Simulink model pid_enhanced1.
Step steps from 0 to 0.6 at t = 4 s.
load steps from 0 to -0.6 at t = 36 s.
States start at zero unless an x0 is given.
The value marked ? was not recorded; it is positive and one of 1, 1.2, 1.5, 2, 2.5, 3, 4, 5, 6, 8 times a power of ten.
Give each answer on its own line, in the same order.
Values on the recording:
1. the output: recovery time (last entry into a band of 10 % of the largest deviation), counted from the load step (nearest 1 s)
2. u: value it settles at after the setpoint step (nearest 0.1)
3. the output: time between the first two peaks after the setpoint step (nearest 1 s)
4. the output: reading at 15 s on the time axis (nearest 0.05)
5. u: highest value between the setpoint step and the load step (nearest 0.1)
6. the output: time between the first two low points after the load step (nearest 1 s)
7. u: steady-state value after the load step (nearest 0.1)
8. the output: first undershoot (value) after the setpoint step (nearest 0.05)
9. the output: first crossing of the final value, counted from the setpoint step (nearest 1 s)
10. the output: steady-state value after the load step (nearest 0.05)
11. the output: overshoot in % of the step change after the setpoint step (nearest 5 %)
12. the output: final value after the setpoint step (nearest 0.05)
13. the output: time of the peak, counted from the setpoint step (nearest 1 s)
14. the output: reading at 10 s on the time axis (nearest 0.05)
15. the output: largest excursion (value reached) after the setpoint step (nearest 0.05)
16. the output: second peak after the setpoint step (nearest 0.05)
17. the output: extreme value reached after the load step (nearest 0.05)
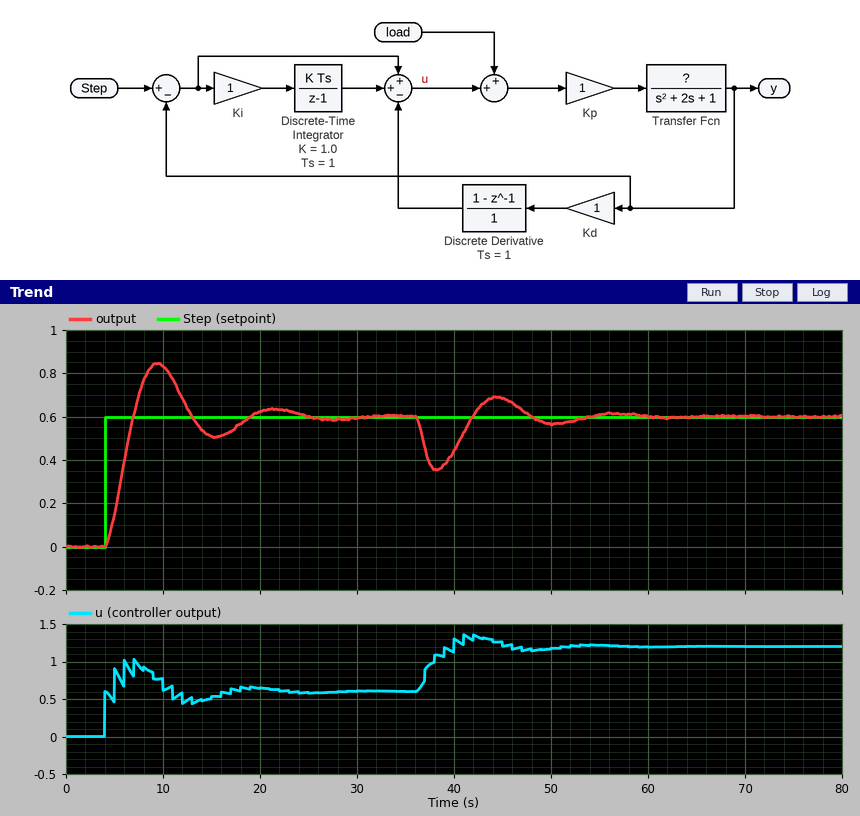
16 s
0.6
12 s
0.50
1.0
12 s
1.2
0.50
3 s
0.60
40 %
0.60
5 s
0.85
0.85
0.65
0.35
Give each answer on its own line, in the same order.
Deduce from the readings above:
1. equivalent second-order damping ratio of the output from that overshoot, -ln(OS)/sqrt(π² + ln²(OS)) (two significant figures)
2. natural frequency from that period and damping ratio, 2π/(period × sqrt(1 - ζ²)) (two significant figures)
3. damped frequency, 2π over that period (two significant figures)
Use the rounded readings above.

0.28
0.55 rad/s
0.52 rad/s
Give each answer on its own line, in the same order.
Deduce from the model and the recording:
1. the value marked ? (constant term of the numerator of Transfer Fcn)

1
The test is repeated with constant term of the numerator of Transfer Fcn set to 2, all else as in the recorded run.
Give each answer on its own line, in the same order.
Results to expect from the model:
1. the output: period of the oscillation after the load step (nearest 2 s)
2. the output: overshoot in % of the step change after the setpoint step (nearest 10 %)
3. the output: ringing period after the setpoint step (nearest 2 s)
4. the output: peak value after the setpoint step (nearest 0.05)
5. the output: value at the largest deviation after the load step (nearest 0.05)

10 s
50 %
10 s
0.90
0.25
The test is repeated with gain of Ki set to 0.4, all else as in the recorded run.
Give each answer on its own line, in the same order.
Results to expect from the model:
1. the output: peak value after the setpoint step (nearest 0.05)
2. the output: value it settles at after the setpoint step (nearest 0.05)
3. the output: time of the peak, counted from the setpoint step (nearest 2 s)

0.65
0.60
10 s
